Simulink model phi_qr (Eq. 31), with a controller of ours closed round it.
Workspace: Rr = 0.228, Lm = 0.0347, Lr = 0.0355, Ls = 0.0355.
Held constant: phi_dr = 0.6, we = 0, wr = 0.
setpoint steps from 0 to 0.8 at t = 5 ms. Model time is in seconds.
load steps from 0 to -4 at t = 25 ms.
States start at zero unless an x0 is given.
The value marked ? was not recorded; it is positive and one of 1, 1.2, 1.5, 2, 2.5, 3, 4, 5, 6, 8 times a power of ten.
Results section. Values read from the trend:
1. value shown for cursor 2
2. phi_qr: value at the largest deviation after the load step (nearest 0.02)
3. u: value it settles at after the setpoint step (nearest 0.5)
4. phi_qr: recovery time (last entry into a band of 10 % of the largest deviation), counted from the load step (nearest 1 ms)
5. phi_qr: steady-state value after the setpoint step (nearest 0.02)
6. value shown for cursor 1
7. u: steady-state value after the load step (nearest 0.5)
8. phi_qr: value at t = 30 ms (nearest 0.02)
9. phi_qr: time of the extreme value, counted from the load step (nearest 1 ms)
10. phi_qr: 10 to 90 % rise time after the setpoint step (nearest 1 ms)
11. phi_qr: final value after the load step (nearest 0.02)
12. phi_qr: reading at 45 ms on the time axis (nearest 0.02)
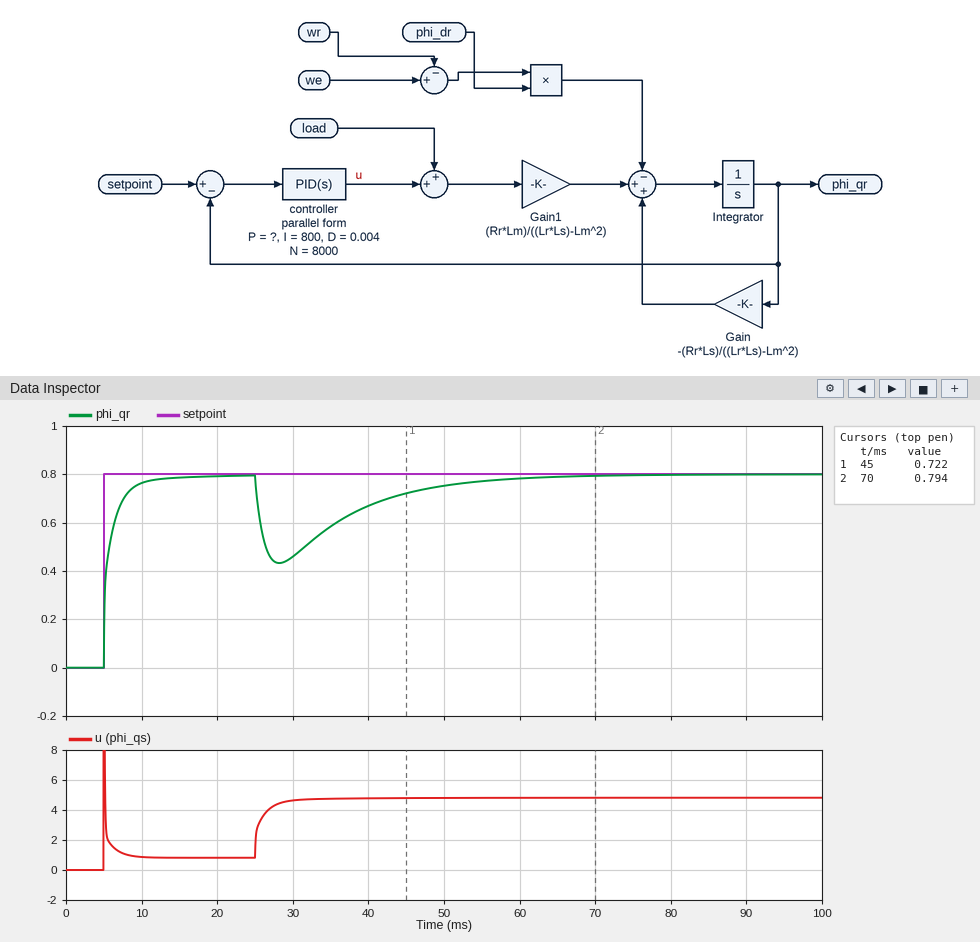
0.794
0.44
1.0
28 ms
0.80
0.722
5.0
0.46
3 ms
3 ms
0.80
0.72
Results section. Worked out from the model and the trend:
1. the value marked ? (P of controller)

8
